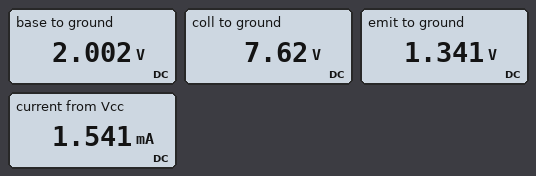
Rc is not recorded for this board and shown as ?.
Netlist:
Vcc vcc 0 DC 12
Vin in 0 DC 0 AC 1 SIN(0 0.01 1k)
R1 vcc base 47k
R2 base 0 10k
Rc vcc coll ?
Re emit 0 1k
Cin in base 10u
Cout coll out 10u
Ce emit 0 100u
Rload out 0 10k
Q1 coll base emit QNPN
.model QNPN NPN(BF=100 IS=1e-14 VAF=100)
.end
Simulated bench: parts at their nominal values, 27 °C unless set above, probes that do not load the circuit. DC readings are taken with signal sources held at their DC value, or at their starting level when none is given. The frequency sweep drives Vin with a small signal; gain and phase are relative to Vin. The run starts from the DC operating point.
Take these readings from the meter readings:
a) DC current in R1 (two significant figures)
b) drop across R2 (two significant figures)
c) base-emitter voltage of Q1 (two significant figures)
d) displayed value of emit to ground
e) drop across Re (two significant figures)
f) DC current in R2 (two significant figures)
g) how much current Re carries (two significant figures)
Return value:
210 µA
2.0 V
660 mV
1.341 V
1.3 V
200 µA
1.3 mA
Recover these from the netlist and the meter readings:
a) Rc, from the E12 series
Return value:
3.3 kΩ
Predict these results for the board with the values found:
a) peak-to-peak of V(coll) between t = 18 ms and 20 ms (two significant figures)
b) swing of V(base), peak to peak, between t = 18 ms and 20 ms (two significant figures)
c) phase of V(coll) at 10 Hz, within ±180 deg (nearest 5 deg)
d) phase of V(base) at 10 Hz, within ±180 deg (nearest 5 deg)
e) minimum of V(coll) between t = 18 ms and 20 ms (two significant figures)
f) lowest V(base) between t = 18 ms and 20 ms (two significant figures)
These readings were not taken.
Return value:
2.4 V
20 mV
-95 deg
10 deg
6.3 V
2.0 V
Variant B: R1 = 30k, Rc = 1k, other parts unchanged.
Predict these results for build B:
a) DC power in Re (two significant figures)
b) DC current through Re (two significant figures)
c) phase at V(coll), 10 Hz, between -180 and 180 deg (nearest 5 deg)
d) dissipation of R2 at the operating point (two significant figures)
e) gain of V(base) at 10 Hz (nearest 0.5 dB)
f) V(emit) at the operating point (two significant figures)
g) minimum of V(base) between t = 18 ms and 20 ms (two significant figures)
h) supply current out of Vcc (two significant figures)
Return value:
4.7 mW
2.2 mA
-90 deg
810 µW
-1.0 dB
2.2 V
2.8 V
2.5 mA
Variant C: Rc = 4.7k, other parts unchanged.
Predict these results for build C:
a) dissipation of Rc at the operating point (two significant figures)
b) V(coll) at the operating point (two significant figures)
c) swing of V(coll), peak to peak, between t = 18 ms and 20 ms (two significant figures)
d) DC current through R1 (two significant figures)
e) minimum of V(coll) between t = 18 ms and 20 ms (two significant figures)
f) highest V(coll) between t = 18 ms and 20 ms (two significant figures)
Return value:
8.3 mW
5.8 V
3.1 V
210 µA
4.1 V
7.2 V
